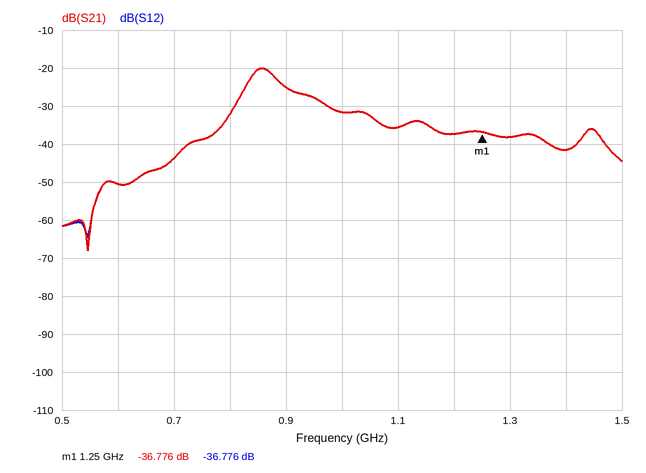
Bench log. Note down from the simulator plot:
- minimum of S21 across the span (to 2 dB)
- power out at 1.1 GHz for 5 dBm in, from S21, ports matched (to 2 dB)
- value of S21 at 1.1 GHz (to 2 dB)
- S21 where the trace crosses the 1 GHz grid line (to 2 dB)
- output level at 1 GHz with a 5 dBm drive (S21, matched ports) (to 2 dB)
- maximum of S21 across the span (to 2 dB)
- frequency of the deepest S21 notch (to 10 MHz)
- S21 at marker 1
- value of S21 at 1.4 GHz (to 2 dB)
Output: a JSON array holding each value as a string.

["-68 dB", "-30 dBm", "-36 dB", "-32 dB", "-26 dBm", "-20 dB", "550 MHz", "-36.776 dB", "-42 dB"]
